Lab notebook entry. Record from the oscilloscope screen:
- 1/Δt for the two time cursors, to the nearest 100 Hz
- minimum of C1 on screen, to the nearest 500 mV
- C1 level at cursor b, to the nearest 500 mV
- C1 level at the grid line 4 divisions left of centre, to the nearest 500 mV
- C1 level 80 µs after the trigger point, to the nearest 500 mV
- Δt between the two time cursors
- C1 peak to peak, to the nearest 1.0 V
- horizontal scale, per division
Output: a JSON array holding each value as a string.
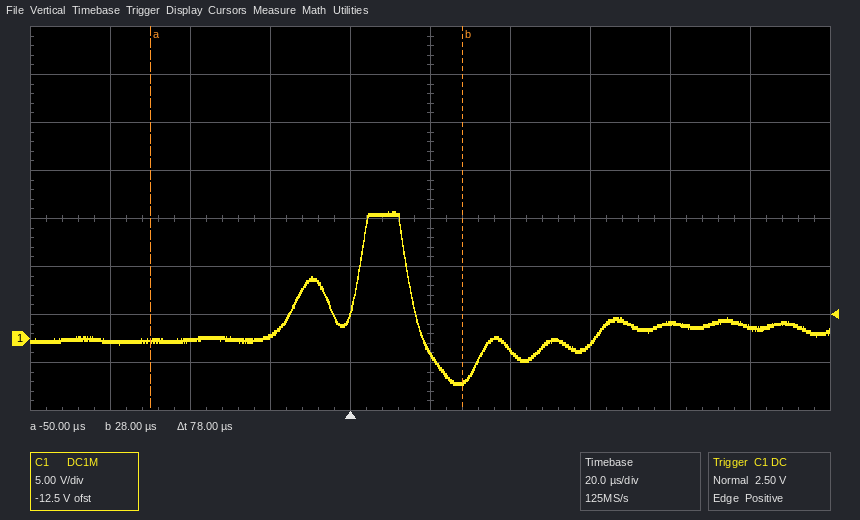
["12.8 kHz", "-5.0 V", "-4.5 V", "-500 mV", "1.5 V", "78 µs", "18.0 V", "20 µs"]
